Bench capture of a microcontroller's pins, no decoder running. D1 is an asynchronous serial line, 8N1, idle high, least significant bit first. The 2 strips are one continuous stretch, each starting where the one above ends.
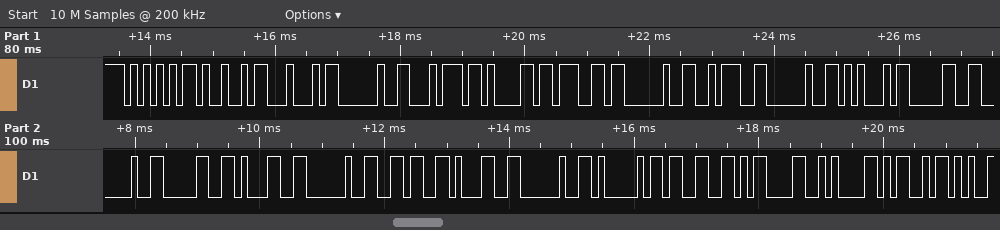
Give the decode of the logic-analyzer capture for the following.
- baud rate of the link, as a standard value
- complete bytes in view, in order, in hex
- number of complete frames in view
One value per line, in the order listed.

9600 baud
55 49 44 20 74 61 67 20 3A 20 45 30 20 30 31 20 36 31 20 41 33 0D 0A 4D
24
